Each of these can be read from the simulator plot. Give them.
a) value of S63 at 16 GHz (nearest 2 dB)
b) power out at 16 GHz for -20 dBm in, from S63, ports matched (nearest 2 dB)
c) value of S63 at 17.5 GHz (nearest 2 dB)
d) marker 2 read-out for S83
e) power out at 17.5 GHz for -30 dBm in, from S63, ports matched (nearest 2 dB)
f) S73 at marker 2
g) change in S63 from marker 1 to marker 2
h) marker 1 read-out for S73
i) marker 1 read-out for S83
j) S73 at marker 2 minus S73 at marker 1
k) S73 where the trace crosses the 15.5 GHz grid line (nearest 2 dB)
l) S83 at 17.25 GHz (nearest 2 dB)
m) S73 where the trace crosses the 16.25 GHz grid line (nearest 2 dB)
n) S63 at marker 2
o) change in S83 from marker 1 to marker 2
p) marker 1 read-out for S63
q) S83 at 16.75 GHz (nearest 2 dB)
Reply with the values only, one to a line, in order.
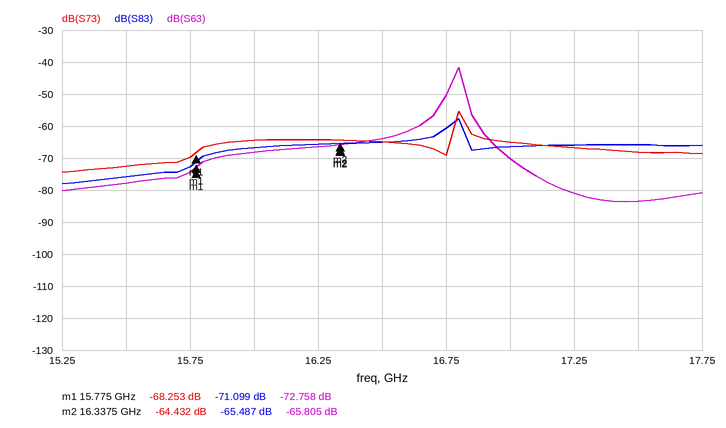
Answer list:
-68 dB
-88 dBm
-84 dB
-65.487 dB
-114 dBm
-64.432 dB
6.953 dB
-68.253 dB
-71.099 dB
3.821 dB
-72 dB
-66 dB
-64 dB
-65.805 dB
5.612 dB
-72.758 dB
-60 dB
